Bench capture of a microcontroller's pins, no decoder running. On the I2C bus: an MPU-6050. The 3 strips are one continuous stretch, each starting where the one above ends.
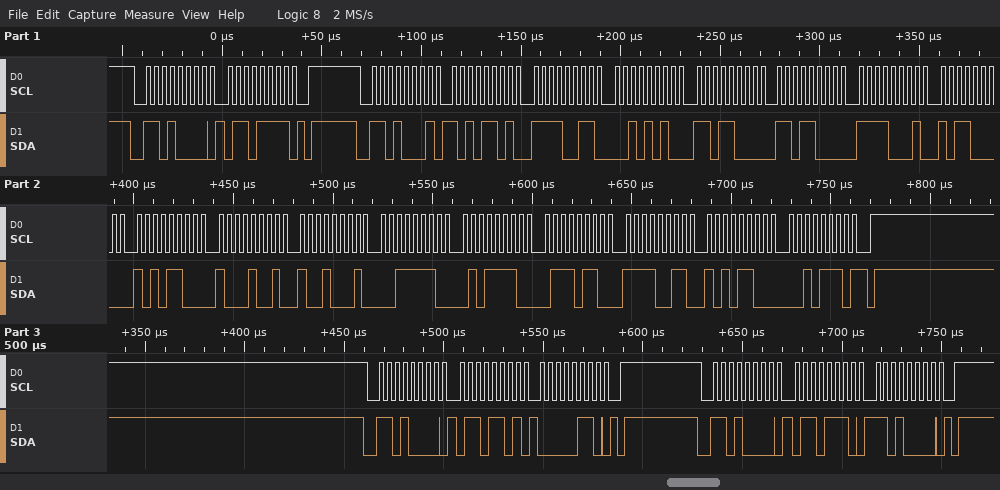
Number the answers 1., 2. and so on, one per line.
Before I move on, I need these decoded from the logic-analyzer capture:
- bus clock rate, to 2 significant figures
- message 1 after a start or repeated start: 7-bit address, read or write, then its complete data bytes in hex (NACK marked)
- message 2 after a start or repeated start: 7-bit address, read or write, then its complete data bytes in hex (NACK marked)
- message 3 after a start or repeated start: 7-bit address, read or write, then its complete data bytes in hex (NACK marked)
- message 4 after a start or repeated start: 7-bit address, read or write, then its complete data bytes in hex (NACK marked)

1. 250 kHz
2. 0x68 write: 6F
3. 0x68 read: AD F3 2A D8 D8 F1 B0 AC 89 91 3E 5E 76 F3 AC 2E NACK
4. 0x68 write: 6D 06
5. 0x68 write: 6E D0
